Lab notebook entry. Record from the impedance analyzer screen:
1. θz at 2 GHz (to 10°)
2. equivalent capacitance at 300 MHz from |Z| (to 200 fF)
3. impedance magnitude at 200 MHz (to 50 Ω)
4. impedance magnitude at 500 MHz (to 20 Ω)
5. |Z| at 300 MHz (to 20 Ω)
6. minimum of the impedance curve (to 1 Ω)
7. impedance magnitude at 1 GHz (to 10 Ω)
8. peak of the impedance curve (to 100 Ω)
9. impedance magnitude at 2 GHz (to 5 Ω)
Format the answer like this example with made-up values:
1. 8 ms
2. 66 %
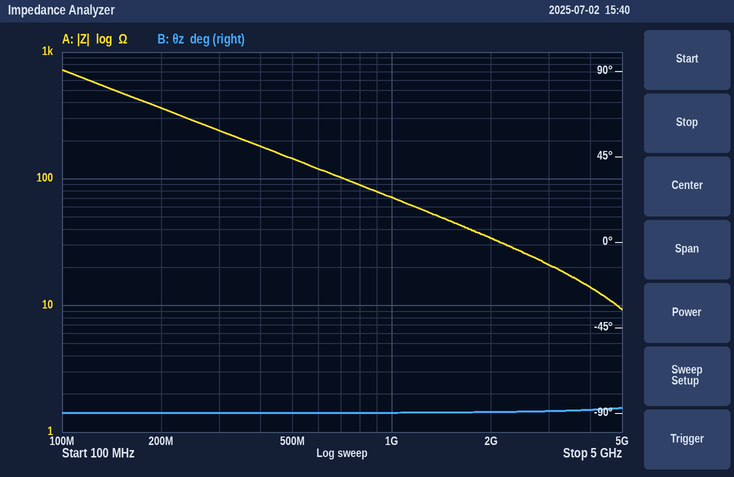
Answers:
1. -90°
2. 2.2 pF
3. 350 Ω
4. 140 Ω
5. 240 Ω
6. 9 Ω
7. 70 Ω
8. 700 Ω
9. 35 Ω
